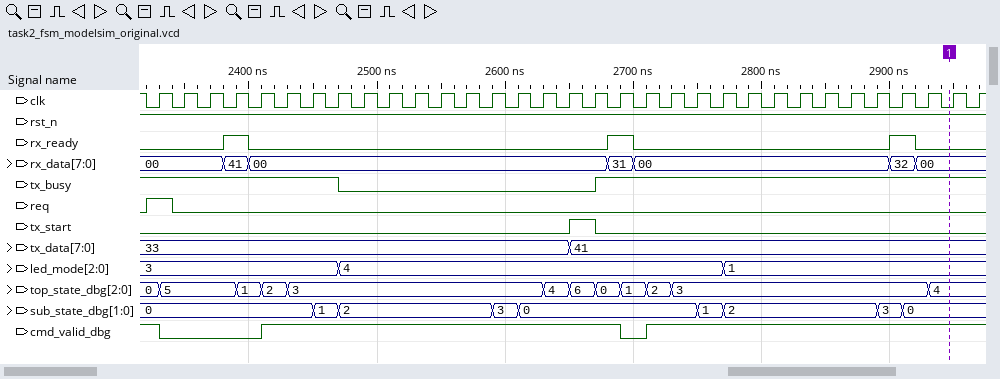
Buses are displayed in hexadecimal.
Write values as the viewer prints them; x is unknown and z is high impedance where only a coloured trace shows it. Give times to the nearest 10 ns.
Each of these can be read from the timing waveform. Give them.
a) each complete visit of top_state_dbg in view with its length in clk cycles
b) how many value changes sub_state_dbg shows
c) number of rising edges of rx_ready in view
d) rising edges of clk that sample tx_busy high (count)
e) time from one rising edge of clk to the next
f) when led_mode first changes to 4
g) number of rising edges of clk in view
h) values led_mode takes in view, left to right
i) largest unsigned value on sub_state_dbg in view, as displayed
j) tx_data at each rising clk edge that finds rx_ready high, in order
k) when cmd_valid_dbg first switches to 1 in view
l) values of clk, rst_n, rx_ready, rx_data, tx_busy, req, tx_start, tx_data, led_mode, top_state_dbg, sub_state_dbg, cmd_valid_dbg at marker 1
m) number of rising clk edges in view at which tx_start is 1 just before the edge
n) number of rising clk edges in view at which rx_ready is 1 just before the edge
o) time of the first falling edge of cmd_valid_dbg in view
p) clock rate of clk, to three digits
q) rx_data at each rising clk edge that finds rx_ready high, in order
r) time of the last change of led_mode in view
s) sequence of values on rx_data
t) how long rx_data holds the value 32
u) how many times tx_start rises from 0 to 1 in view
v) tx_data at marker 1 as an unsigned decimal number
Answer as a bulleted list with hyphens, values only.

- 5: 3, 1: 1, 2: 1, 3: 10, 4: 1, 6: 1, 0: 1, 1: 1, 2: 1, 3: 10
- 8
- 3
- 23
- 20 ns
- 2470 ns
- 33
- 3, 4, 1
- 3
- 33, 41, 41
- 2410 ns
- clk=0, rst_n=1, rx_ready=0, rx_data=00, tx_busy=1, req=0, tx_start=0, tx_data=41, led_mode=1, top_state_dbg=4, sub_state_dbg=0, cmd_valid_dbg=1
- 1
- 3
- 2330 ns
- 50.0 MHz
- 41, 31, 32
- 2770 ns
- 00, 41, 00, 31, 00, 32, 00
- 20 ns
- 1
- 65
